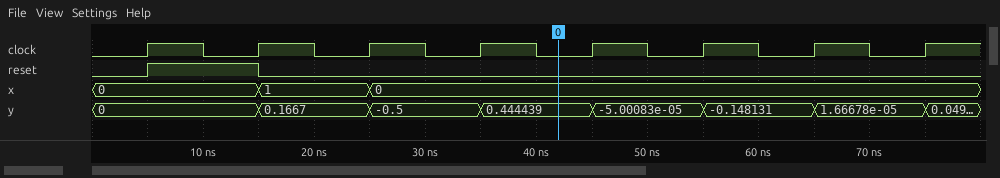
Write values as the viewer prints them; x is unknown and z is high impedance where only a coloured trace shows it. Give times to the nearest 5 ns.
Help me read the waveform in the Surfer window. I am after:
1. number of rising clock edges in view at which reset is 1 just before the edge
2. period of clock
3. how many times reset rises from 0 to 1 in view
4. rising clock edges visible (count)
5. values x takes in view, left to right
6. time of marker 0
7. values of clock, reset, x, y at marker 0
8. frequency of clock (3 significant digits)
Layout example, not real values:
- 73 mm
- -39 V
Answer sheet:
- 1
- 10 ns
- 1
- 8
- 0, 1, 0
- 40 ns
- clock=0, reset=0, x=0, y=0.444439
- 100 MHz
